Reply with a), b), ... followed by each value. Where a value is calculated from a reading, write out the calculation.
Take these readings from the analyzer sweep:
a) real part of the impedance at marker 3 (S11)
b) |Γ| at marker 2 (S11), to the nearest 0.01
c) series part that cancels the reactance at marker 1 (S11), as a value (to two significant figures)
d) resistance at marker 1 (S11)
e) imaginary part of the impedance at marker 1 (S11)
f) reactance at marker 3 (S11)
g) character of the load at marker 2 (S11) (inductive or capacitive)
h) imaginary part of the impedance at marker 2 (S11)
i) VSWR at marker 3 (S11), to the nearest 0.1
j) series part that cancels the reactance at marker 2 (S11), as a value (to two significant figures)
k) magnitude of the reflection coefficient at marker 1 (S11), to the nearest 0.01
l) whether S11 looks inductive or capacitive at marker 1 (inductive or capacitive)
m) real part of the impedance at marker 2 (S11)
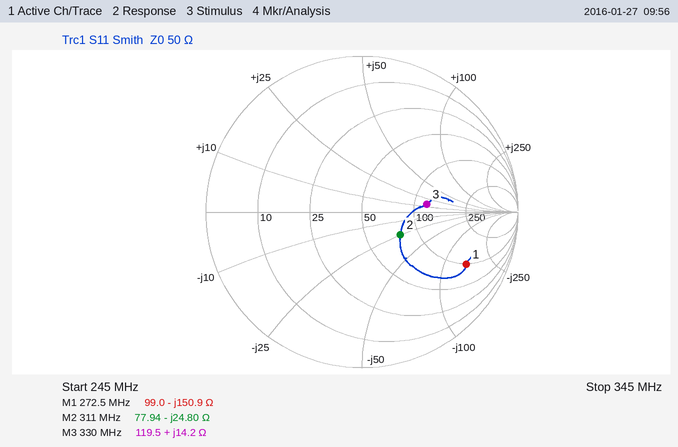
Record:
a) 119.5 Ω
b) 0.29
c) L = 150.9 Ω/(2π × 272.5 MHz) ≈ 88 nH
d) 99.0 Ω
e) -150.9 Ω
f) +14.2 Ω
g) capacitive
h) -24.80 Ω
i) 2.4
j) L = 24.8 Ω/(2π × 311 MHz) ≈ 13 nH
k) 0.75
l) capacitive
m) 77.94 Ω
